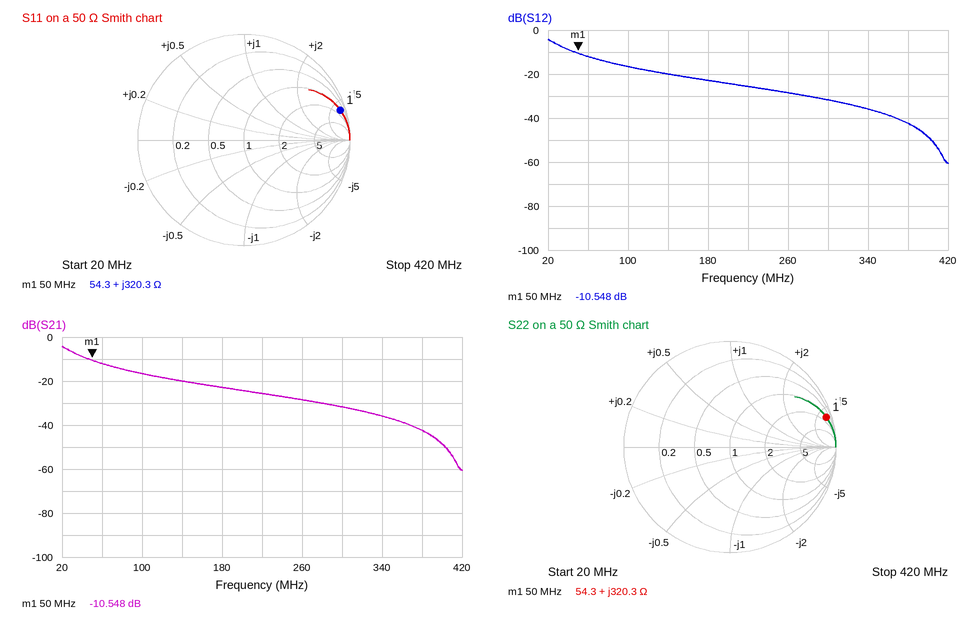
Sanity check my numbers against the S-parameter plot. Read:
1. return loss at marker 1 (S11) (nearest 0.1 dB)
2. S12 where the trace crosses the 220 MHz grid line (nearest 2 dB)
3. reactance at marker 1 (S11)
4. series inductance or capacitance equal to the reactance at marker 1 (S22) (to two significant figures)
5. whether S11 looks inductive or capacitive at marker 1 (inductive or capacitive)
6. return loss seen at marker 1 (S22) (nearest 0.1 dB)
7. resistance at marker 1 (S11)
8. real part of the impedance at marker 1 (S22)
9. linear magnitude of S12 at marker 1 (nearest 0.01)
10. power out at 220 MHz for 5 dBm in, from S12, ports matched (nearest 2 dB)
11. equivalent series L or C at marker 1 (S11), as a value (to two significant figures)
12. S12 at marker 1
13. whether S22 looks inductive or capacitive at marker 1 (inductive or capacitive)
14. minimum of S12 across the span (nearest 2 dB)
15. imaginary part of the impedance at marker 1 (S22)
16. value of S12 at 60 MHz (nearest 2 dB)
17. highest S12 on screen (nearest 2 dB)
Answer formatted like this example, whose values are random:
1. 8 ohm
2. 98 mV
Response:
1. 0.4 dB
2. -26 dB
3. +320.3 Ω
4. 1.0 µH
5. inductive
6. 0.4 dB
7. 54.3 Ω
8. 54.3 Ω
9. 0.30
10. -20 dBm
11. 1.0 µH
12. -10.548 dB
13. inductive
14. -60 dB
15. +320.3 Ω
16. -12 dB
17. -4 dB
